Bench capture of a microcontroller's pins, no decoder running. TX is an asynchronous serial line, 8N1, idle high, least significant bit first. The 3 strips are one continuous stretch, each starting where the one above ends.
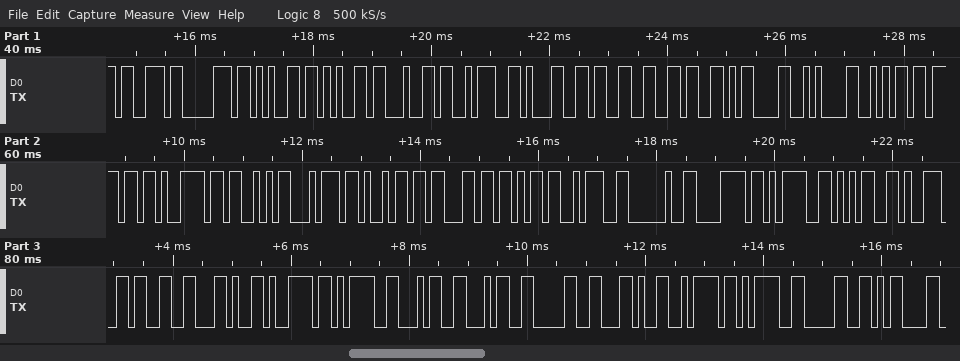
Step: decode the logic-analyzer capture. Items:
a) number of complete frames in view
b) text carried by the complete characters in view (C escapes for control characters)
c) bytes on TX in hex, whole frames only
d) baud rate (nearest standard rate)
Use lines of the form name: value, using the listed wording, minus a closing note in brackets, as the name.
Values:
number of complete frames in view: 37
text carried by the complete characters in view: "speed:136\r\njoyStick: x=593,y=440,z=0\r"
bytes on TX in hex, whole frames only: 0x73 0x70 0x65 0x65 0x64 0x3A 0x31 0x33 0x36 0x0D 0x0A 0x6A 0x6F 0x79 0x53 0x74 0x69 0x63 0x6B 0x3A 0x20 0x78 0x3D 0x35 0x39 0x33 0x2C 0x79 0x3D 0x34 0x34 0x30 0x2C 0x7A 0x3D 0x30 0x0D
baud rate: 9600 baud
